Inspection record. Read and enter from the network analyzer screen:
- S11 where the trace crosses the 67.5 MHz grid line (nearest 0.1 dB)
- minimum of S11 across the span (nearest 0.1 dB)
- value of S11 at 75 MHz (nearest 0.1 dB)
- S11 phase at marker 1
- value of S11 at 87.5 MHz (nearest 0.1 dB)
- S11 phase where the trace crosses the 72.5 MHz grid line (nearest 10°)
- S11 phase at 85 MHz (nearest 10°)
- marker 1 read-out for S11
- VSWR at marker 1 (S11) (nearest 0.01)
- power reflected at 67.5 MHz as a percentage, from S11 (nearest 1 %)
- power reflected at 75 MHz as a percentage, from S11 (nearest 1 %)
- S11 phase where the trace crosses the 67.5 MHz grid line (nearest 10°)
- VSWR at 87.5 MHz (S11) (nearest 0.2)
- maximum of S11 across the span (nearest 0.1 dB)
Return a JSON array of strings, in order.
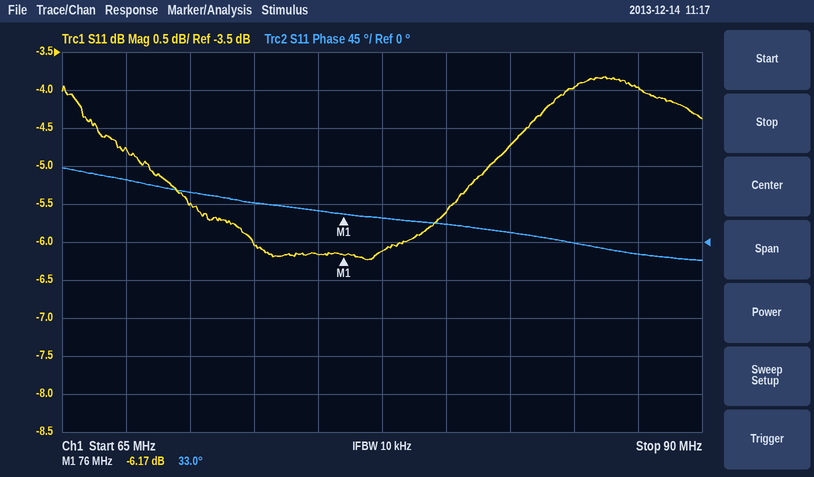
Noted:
["-4.8 dB", "-6.2 dB", "-6.2 dB", "33.0°", "-4.0 dB", "50°", "0°", "-6.17 dB", "2.93", "33 %", "24 %", "70°", "4.4", "-3.8 dB"]
